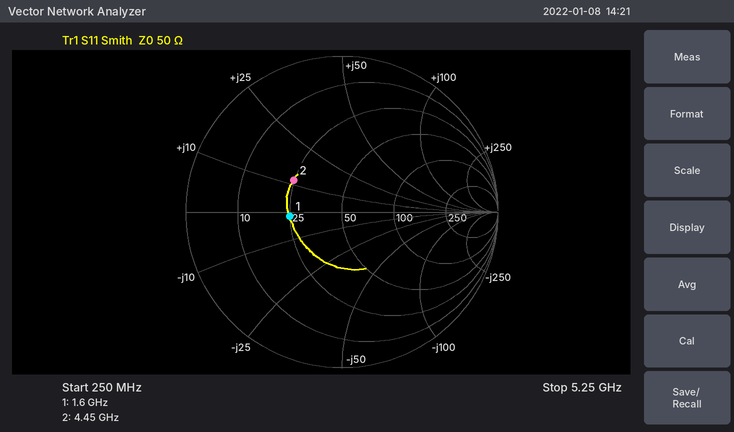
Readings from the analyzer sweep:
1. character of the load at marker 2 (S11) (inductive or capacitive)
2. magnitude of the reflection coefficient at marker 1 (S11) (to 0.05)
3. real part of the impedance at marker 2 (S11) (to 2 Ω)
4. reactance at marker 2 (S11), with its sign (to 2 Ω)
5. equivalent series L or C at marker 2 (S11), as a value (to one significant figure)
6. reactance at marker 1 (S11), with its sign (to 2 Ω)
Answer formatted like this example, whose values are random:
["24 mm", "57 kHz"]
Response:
["inductive", "0.35", "24 Ω", "+12 Ω", "400 pH", "-2 Ω"]
